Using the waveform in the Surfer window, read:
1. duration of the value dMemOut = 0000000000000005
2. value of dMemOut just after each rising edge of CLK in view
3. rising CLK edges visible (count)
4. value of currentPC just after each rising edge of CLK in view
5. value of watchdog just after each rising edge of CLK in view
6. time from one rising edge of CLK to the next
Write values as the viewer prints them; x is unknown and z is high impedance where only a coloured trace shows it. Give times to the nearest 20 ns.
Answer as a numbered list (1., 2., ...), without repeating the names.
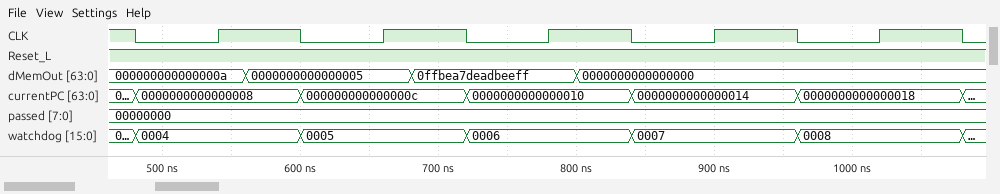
1. 120 ns
2. 000000000000000a, 0000000000000005, 0ffbea7deadbeeff, 0000000000000000, 0000000000000000
3. 5
4. 0000000000000008, 000000000000000c, 0000000000000010, 0000000000000014, 0000000000000018
5. 0004, 0005, 0006, 0007, 0008
6. 120 ns
